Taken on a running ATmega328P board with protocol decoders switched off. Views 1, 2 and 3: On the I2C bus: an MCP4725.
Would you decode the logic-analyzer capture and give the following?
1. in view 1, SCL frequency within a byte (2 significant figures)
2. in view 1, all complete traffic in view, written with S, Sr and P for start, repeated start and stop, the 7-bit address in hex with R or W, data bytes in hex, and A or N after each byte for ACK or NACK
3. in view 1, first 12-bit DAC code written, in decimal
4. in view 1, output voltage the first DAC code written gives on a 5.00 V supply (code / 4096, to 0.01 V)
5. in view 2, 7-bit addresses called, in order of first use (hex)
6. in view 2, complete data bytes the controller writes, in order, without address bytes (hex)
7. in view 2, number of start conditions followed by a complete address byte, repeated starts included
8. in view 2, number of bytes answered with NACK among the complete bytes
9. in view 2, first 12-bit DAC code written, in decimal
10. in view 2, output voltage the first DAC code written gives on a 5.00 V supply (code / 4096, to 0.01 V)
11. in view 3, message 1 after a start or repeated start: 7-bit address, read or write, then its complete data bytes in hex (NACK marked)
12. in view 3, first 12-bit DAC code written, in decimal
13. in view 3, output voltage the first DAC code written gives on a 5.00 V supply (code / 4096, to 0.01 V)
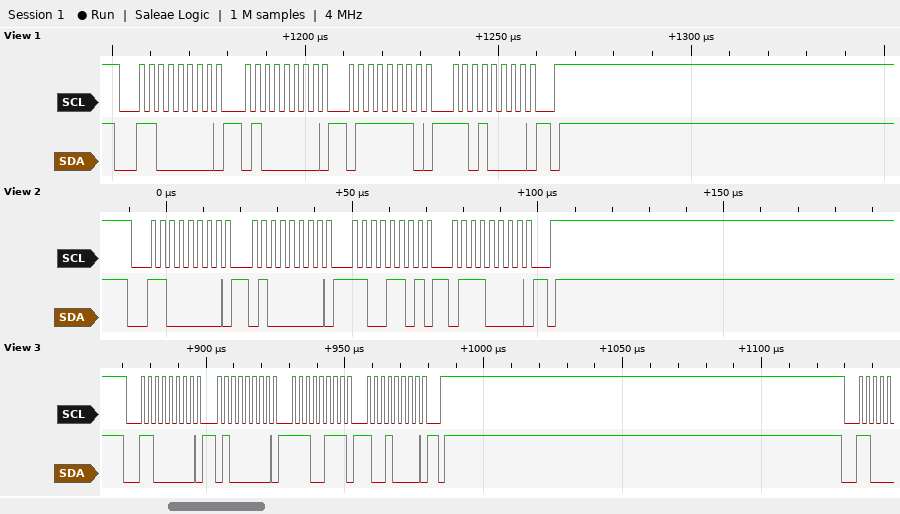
400 kHz
S 60W A 40 A 7E A D0 A P
2029
2.48 V
0x60
40 CD 70
1
0
3287
4.01 V
0x60 write: 40 E7 90
3705
4.52 V
